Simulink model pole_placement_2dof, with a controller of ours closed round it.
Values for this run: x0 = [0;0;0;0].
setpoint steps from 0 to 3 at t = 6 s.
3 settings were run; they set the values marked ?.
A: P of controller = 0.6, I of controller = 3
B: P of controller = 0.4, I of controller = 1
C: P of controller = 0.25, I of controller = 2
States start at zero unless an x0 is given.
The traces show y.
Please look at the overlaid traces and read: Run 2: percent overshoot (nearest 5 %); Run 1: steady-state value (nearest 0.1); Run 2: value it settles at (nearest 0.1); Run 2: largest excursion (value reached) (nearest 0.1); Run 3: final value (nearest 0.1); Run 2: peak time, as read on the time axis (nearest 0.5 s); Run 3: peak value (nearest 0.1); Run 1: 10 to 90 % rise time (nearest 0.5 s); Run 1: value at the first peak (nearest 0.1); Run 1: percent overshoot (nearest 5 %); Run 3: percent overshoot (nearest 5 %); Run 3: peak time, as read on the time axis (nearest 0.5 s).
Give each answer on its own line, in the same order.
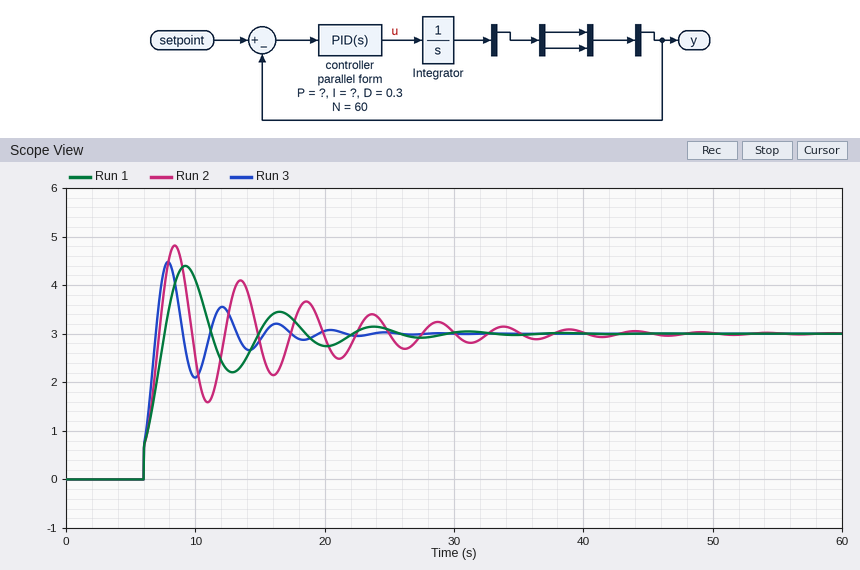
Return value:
60 %
3.0
3.0
4.8
3.0
8.5 s
4.5
1.5 s
4.4
45 %
50 %
8.0 s
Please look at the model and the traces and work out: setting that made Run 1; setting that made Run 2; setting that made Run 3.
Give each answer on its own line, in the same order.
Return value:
B
C
A
